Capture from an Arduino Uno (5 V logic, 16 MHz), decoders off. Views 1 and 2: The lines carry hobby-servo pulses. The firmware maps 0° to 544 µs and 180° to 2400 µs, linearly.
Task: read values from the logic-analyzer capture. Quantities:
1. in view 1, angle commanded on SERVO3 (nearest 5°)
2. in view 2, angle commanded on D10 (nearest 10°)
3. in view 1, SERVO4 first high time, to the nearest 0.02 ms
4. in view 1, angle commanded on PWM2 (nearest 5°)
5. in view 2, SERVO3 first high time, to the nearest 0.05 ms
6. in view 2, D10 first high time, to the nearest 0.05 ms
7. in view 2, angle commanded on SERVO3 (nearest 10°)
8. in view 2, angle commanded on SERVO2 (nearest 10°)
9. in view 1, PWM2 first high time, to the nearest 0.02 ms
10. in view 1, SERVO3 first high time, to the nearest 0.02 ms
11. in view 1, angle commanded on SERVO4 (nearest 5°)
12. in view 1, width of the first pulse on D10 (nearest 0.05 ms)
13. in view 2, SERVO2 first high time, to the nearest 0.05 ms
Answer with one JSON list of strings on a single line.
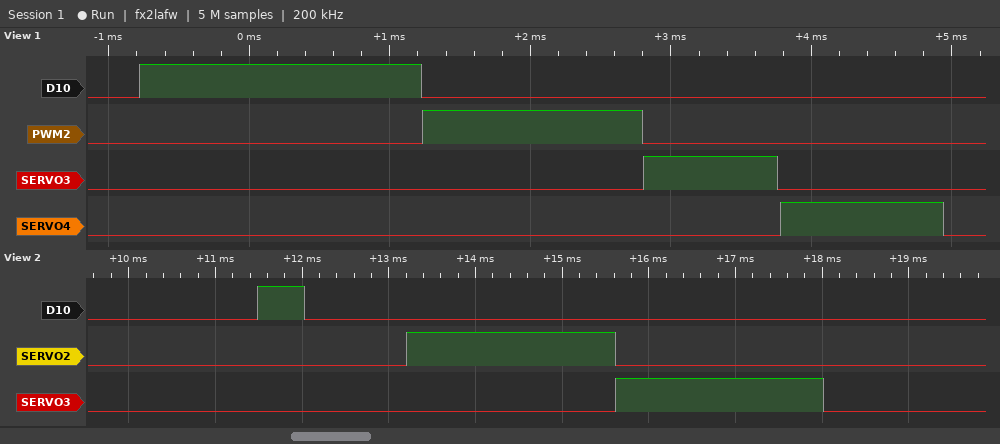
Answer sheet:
["40°", "0°", "1.16 ms", "100°", "2.40 ms", "0.55 ms", "180°", "180°", "1.56 ms", "0.96 ms", "60°", "2.00 ms", "2.40 ms"]
